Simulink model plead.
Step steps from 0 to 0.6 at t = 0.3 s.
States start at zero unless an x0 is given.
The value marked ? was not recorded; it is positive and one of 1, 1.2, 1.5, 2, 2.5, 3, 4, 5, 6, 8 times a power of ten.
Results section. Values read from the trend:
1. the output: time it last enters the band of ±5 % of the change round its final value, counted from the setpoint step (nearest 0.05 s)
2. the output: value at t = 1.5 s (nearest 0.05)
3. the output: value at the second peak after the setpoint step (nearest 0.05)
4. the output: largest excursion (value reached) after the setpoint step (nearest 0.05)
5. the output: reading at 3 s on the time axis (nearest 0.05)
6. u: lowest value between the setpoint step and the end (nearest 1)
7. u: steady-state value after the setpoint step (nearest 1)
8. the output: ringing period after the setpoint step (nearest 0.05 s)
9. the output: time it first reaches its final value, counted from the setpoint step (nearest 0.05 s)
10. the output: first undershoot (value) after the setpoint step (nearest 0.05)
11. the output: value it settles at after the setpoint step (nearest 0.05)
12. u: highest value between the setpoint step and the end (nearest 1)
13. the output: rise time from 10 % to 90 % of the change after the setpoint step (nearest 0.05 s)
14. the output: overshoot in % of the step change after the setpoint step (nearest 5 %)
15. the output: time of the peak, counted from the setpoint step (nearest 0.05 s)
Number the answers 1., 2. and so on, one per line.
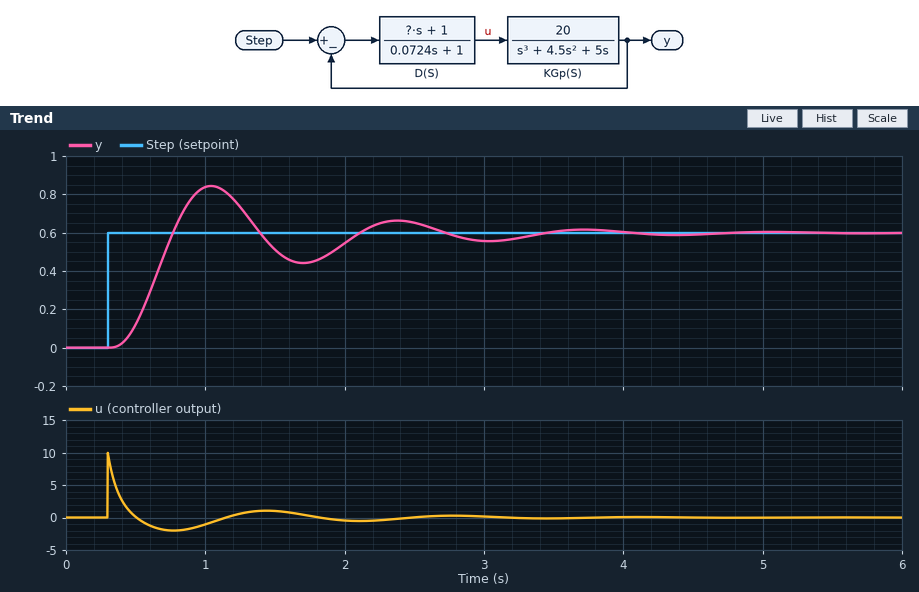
1. 2.95 s
2. 0.50
3. 0.65
4. 0.85
5. 0.55
6. -2
7. 0
8. 1.35 s
9. 0.45 s
10. 0.45
11. 0.60
12. 10
13. 0.30 s
14. 40 %
15. 0.75 s
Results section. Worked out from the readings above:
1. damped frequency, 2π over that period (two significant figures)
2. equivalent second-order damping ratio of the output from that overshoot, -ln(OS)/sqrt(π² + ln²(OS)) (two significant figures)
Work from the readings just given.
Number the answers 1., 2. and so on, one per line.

1. 4.7 rad/s
2. 0.28
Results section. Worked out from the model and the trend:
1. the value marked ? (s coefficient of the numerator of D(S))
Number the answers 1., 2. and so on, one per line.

1. 1.2
